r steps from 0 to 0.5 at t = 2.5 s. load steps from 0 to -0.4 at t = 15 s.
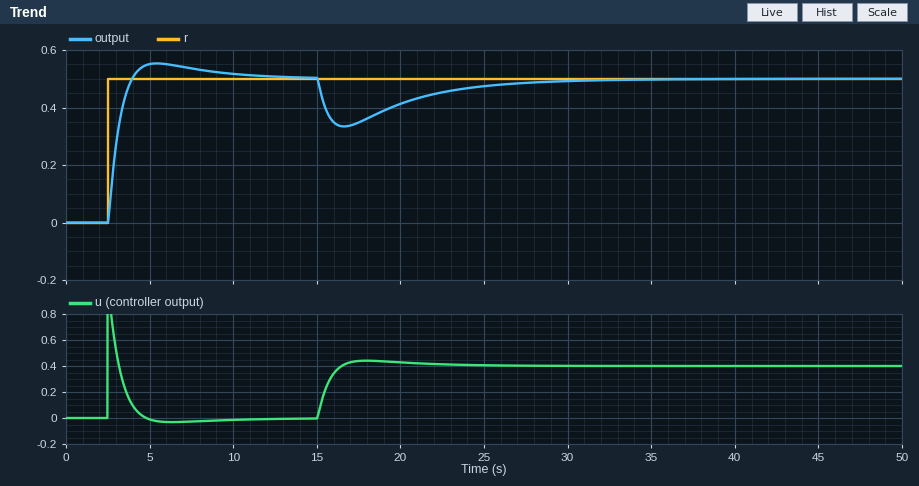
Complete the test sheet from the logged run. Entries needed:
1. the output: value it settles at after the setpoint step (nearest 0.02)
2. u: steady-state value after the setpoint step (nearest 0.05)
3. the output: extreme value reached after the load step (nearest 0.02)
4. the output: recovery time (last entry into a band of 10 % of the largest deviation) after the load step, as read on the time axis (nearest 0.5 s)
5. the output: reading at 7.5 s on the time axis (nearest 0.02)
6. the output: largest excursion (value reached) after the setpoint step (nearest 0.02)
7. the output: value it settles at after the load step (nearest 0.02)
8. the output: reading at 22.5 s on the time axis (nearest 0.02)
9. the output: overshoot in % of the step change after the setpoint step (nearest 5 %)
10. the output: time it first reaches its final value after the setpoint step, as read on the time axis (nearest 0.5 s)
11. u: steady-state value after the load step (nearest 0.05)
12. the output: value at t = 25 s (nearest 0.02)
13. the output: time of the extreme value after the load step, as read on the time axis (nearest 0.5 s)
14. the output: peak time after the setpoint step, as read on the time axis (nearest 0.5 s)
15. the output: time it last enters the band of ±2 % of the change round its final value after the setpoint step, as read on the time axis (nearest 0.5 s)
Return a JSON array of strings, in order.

["0.50", "0.00", "0.34", "27.0 s", "0.54", "0.56", "0.50", "0.46", "10 %", "4.0 s", "0.40", "0.48", "16.5 s", "5.5 s", "11.5 s"]
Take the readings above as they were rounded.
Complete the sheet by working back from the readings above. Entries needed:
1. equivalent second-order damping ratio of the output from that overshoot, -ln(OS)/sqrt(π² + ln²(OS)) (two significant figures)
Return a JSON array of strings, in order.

["0.59"]
